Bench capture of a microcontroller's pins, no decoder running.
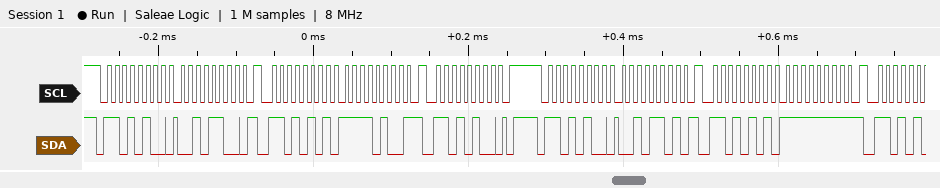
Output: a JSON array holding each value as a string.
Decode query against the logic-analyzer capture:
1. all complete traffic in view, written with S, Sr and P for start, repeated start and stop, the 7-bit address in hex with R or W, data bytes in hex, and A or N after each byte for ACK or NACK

["S 6AW A 2C A Sr 6AR A F4 N Sr 6AW A P S 6AW A 2D A Sr 6AR A FF N"]
